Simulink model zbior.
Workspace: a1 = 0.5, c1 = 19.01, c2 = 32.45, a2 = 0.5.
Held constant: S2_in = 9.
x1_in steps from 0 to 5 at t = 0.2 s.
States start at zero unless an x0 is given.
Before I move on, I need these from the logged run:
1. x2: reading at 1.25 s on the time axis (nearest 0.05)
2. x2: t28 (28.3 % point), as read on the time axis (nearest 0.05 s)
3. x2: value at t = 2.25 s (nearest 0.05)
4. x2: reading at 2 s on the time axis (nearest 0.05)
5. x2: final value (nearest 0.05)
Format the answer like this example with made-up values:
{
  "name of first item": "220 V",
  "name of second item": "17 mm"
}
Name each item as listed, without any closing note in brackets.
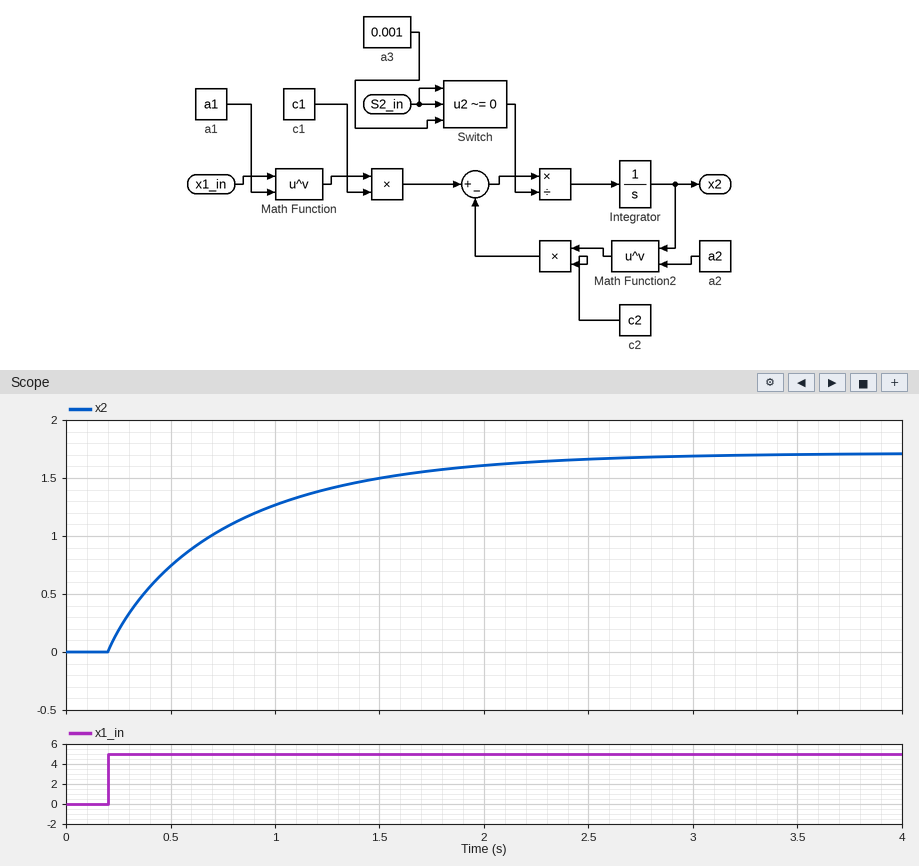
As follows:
{
  "x2: reading at 1.25 s on the time axis": "1.40",
  "x2: t28 (28.3 % point), as read on the time axis": "0.35 s",
  "x2: value at t = 2.25 s": "1.65",
  "x2: reading at 2 s on the time axis": "1.60",
  "x2: final value": "1.70"
}
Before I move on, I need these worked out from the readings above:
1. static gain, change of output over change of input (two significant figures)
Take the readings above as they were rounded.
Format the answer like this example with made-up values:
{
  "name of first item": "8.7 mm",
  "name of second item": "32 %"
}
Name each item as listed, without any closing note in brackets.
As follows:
{
  "static gain, change of output over change of input": "0.34"
}
